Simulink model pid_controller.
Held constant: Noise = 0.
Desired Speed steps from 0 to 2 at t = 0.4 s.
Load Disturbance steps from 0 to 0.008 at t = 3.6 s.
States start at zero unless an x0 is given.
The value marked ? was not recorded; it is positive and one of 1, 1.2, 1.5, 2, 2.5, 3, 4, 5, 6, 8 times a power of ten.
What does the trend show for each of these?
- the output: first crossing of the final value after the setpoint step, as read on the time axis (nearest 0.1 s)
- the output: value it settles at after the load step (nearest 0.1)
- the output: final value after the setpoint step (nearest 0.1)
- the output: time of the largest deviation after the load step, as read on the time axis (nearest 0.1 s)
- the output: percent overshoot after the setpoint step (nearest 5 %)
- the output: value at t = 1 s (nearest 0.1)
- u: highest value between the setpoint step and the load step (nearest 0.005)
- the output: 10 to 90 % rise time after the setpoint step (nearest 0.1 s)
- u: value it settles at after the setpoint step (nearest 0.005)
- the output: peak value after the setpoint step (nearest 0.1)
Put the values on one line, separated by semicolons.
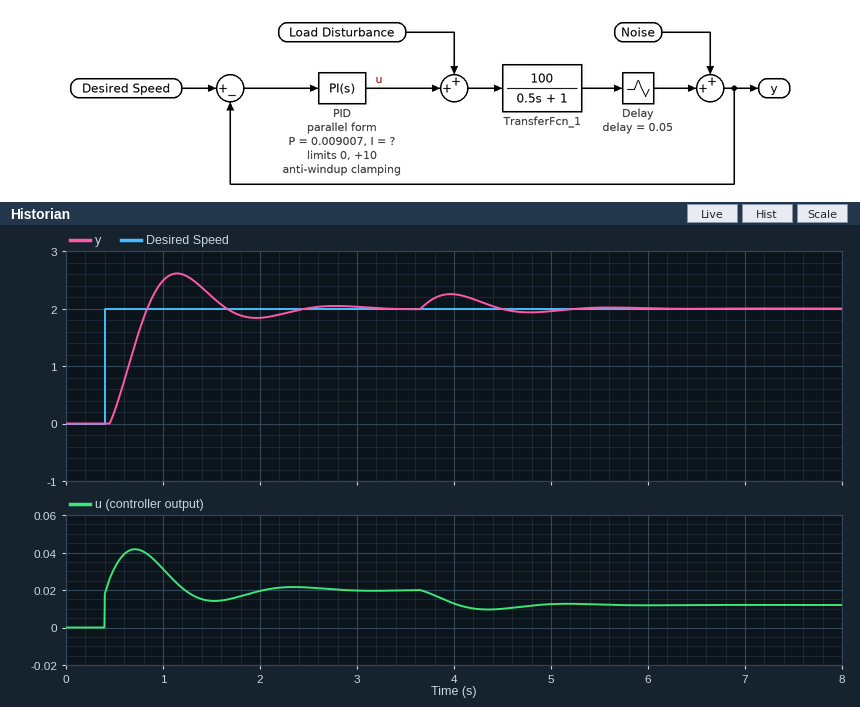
0.8 s; 2.0; 2.0; 4.0 s; 30 %; 2.5; 0.040; 0.3 s; 0.020; 2.6
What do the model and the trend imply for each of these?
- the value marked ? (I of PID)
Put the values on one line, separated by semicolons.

0.08
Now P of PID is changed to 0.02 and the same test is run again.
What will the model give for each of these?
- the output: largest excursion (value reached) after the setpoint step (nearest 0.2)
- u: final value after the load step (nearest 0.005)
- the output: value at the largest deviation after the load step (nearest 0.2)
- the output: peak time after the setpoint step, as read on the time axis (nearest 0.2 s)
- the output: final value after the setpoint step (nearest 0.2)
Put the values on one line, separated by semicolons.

2.2; 0.010; 2.2; 1.0 s; 2.0
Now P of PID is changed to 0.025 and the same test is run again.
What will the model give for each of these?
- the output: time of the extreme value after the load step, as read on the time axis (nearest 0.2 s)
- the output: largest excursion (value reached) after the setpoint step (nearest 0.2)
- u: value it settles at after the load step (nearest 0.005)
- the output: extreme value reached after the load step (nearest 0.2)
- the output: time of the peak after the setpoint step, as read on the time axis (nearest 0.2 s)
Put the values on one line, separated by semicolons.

3.8 s; 2.2; 0.010; 2.2; 1.0 s
